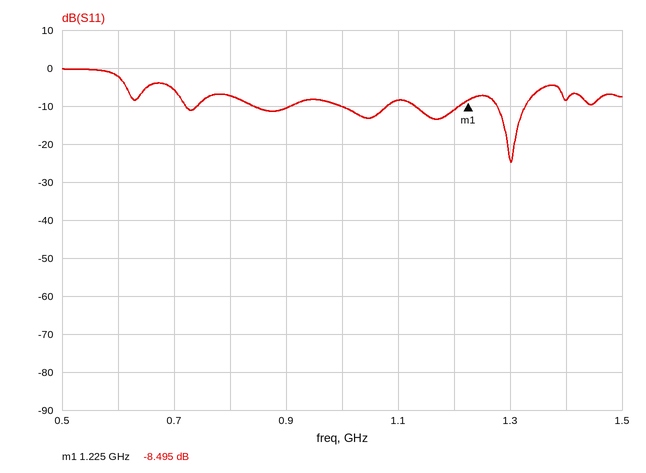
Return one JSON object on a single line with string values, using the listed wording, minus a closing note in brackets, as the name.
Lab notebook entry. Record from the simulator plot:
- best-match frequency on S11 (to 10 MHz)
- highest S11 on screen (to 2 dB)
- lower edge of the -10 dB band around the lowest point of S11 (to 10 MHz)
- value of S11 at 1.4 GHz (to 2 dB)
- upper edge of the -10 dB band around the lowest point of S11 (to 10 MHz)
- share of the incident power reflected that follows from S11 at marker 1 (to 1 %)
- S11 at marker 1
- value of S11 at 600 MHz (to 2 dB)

{"best-match frequency on S11": "1.30 GHz", "highest S11 on screen": "0 dB", "lower edge of the -10 dB band around the lowest point of S11": "1.28 GHz", "value of S11 at 1.4 GHz": "-8 dB", "upper edge of the -10 dB band around the lowest point of S11": "1.33 GHz", "share of the incident power reflected that follows from S11 at marker 1": "14 %", "S11 at marker 1": "-8.495 dB", "value of S11 at 600 MHz": "-2 dB"}
